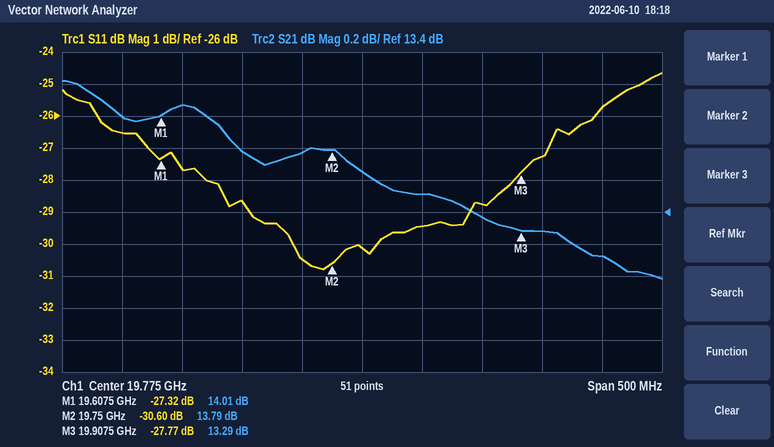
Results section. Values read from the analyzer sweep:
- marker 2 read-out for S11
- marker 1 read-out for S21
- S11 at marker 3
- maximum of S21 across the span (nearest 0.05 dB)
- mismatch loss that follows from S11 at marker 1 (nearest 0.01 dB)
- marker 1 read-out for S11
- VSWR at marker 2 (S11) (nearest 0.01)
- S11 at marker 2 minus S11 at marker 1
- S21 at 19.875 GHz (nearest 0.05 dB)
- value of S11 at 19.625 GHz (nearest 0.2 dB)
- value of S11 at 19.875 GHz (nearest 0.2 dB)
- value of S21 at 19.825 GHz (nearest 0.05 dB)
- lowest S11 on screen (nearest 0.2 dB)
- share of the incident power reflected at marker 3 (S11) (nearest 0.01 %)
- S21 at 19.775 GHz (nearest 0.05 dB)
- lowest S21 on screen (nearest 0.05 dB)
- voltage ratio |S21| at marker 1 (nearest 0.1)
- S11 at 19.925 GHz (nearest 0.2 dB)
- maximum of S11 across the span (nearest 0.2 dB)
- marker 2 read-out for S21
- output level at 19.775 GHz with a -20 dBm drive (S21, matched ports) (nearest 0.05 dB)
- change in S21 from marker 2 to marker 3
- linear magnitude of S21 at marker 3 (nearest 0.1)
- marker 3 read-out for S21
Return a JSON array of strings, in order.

["-30.60 dB", "14.01 dB", "-27.77 dB", "14.20 dB", "0.01 dB", "-27.32 dB", "1.06", "-3.28 dB", "13.35 dB", "-27.6 dB", "-28.8 dB", "13.50 dB", "-30.8 dB", "0.17 %", "13.65 dB", "13.00 dB", "5.0", "-27.2 dB", "-24.6 dB", "13.79 dB", "-6.35 dBm", "-0.50 dB", "4.6", "13.29 dB"]
